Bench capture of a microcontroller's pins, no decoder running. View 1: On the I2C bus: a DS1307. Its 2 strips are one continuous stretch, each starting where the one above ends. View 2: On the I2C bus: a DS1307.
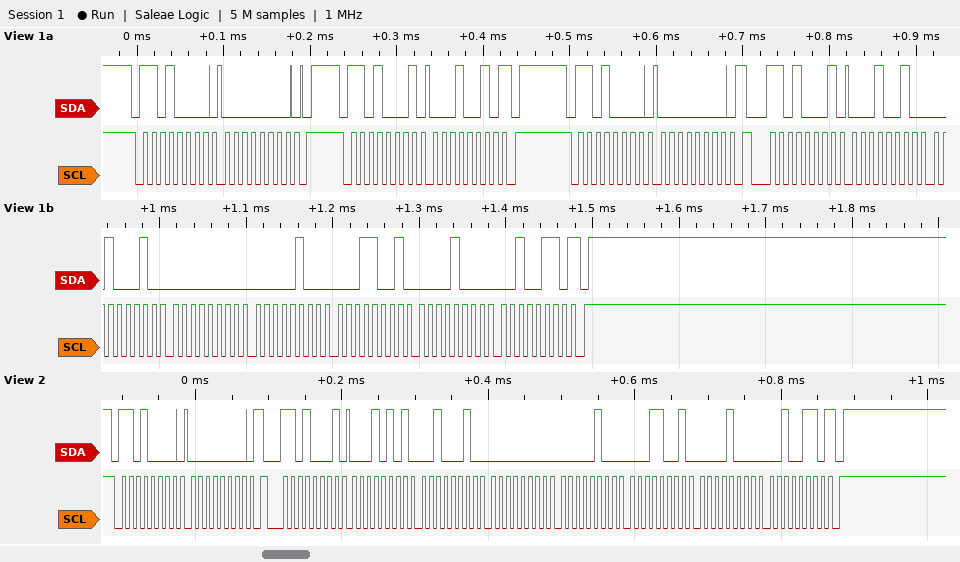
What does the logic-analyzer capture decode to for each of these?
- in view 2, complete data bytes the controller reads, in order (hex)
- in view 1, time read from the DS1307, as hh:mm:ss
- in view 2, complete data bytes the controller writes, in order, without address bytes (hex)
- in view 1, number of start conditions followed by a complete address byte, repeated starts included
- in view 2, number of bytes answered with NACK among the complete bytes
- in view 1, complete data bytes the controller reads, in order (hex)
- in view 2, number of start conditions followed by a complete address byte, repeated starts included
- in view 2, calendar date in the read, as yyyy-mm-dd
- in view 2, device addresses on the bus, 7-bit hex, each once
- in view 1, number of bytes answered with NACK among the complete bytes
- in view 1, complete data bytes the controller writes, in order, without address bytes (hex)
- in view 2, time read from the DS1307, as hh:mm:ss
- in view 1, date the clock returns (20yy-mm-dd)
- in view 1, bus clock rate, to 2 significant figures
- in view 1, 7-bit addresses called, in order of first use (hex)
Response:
15 22 00 04 19 08 26
00:22:12
00
4
1
12 12 22 00 04 19 08 26
2
2026-08-19
0x68
2
00 00
00:22:15
2026-08-19
100 kHz
0x68
